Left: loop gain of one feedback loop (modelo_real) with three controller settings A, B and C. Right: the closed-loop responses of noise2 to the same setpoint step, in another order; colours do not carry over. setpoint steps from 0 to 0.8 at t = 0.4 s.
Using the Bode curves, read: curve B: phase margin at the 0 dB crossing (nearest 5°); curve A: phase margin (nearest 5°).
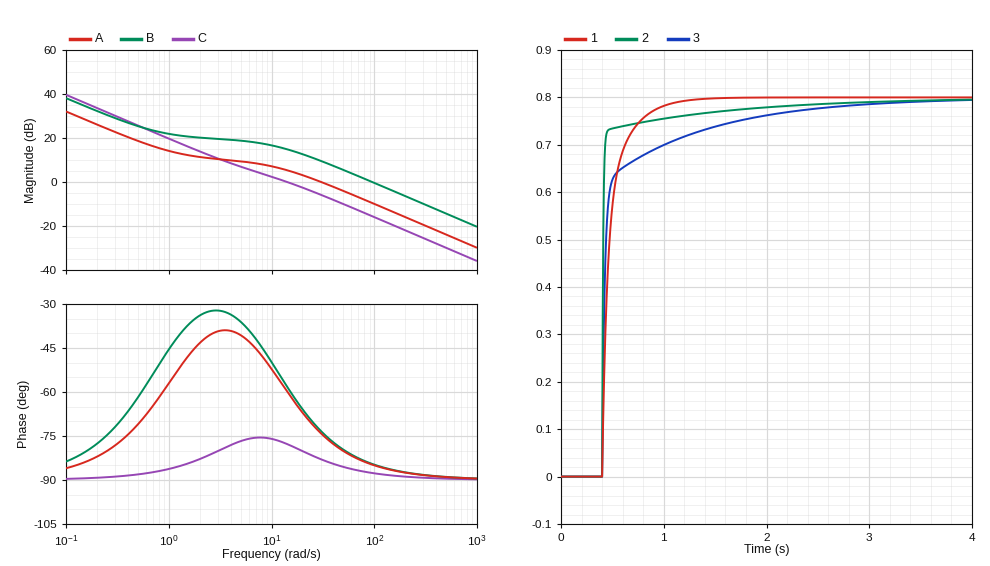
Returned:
95°
105°
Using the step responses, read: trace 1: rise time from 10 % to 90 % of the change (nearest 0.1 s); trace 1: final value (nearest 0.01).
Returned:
0.3 s
0.80
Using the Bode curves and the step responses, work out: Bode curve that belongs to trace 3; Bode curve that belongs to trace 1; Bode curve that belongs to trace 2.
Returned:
A
C
B
